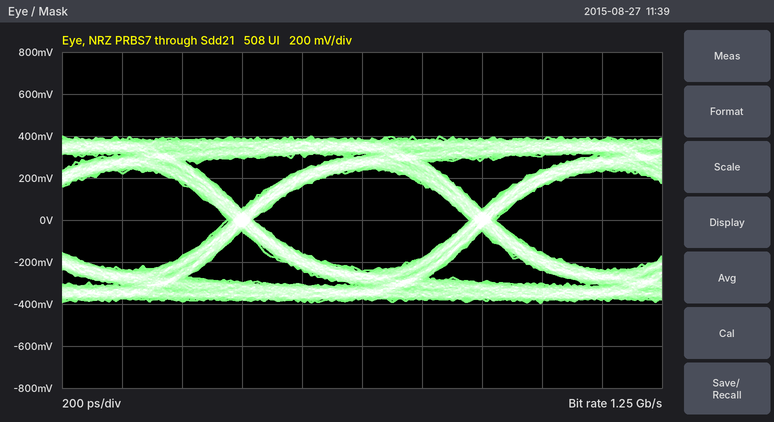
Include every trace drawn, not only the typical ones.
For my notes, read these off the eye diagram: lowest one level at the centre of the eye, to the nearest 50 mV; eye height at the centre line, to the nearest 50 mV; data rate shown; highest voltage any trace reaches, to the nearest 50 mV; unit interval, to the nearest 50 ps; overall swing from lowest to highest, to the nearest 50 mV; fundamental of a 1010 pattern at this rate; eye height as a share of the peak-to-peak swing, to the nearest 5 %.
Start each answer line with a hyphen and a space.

- 250 mV
- 500 mV
- 1.25 Gb/s
- 400 mV
- 800 ps
- 800 mV
- 625 MHz
- 60 %
